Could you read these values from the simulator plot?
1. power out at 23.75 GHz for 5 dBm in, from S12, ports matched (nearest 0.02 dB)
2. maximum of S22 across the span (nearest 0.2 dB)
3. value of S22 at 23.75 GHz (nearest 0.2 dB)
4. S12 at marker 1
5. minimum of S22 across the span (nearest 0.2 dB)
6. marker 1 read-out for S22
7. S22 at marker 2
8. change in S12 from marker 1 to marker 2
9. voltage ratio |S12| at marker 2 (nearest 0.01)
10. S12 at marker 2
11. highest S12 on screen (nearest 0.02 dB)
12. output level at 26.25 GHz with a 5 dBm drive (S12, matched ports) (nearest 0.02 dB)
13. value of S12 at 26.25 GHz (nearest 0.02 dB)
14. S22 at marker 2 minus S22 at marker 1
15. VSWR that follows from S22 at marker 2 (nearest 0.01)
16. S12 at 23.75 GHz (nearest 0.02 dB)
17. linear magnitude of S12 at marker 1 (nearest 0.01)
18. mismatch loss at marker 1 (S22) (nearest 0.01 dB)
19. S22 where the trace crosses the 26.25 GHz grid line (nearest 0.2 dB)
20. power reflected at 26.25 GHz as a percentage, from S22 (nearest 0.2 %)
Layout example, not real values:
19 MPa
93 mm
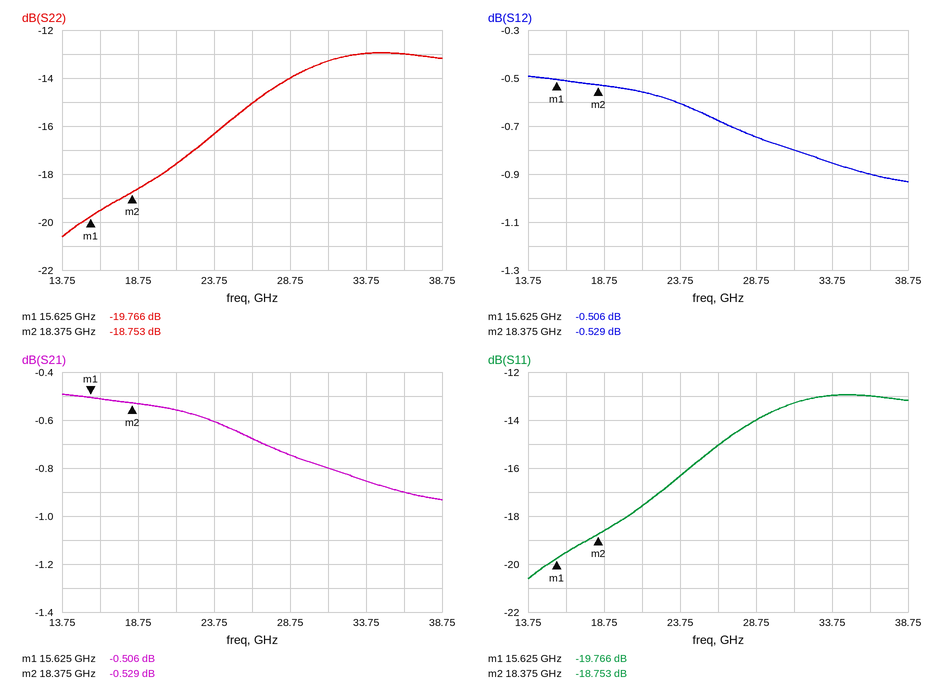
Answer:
4.40 dBm
-13.0 dB
-16.4 dB
-0.506 dB
-20.6 dB
-19.766 dB
-18.753 dB
-0.023 dB
0.94
-0.529 dB
-0.50 dB
4.32 dBm
-0.68 dB
1.013 dB
1.26
-0.60 dB
0.94
0.05 dB
-15.0 dB
3.2 %
